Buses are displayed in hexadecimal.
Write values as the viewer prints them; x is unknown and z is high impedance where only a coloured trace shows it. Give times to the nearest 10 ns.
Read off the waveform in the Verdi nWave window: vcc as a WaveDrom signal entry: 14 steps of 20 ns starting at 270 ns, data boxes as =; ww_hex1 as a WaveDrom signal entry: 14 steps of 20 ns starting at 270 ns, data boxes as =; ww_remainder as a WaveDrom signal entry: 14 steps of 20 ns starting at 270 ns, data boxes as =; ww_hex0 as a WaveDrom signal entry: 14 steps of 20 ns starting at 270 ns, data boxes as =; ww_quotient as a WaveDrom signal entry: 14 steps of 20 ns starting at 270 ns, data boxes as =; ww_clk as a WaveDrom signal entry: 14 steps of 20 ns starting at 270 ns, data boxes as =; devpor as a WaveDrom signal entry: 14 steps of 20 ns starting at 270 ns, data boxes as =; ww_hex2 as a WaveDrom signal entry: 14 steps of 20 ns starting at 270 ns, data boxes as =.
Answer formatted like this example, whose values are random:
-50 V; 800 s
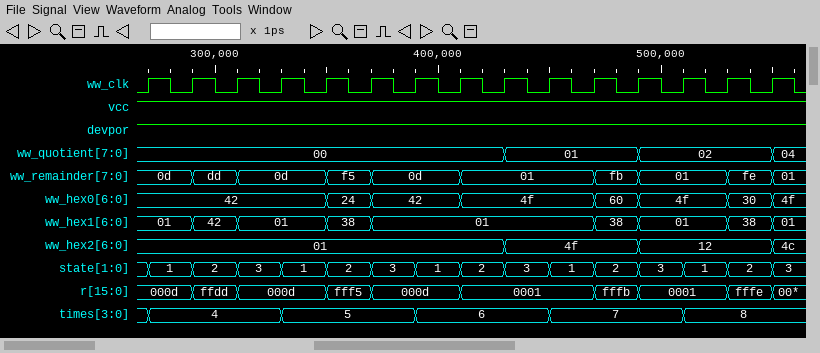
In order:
{name: 'vcc', wave: '1.............'}; {name: 'ww_hex1', wave: '===.==....==.=', data: '01 42 01 38 01 38 01 38'}; {name: 'ww_remainder', wave: '===.==.=..==.=', data: '0d dd 0d f5 0d 01 fb 01 fe'}; {name: 'ww_hex0', wave: '=...==.=..==.=', data: '42 24 42 4f 60 4f 30'}; {name: 'ww_quotient', wave: '=.......=..=..', data: '00 01 02'}; {name: 'ww_clk', wave: 'p.............'}; {name: 'devpor', wave: '1.............'}; {name: 'ww_hex2', wave: '=.......=..=..', data: '01 4f 12'}
